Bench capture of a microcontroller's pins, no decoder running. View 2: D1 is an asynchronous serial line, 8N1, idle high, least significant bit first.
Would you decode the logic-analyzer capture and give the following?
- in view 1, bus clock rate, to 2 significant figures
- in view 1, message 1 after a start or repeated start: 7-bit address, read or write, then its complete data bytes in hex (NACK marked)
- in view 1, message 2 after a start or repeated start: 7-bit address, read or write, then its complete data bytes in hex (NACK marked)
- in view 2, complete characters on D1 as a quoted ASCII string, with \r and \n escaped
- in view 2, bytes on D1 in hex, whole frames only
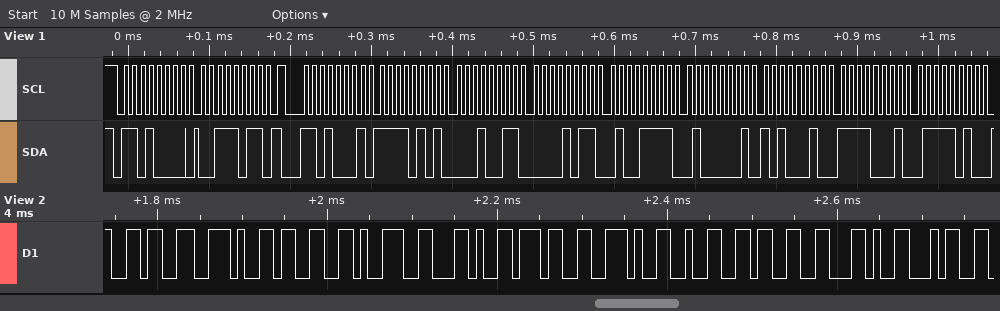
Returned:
100 kHz
0x68 write: 3B
0x68 read: F5 13 0B 4F 41 A2 F1 7A
"6.39,7.23,4"
36 2E 33 39 2C 37 2E 32 33 2C 34
